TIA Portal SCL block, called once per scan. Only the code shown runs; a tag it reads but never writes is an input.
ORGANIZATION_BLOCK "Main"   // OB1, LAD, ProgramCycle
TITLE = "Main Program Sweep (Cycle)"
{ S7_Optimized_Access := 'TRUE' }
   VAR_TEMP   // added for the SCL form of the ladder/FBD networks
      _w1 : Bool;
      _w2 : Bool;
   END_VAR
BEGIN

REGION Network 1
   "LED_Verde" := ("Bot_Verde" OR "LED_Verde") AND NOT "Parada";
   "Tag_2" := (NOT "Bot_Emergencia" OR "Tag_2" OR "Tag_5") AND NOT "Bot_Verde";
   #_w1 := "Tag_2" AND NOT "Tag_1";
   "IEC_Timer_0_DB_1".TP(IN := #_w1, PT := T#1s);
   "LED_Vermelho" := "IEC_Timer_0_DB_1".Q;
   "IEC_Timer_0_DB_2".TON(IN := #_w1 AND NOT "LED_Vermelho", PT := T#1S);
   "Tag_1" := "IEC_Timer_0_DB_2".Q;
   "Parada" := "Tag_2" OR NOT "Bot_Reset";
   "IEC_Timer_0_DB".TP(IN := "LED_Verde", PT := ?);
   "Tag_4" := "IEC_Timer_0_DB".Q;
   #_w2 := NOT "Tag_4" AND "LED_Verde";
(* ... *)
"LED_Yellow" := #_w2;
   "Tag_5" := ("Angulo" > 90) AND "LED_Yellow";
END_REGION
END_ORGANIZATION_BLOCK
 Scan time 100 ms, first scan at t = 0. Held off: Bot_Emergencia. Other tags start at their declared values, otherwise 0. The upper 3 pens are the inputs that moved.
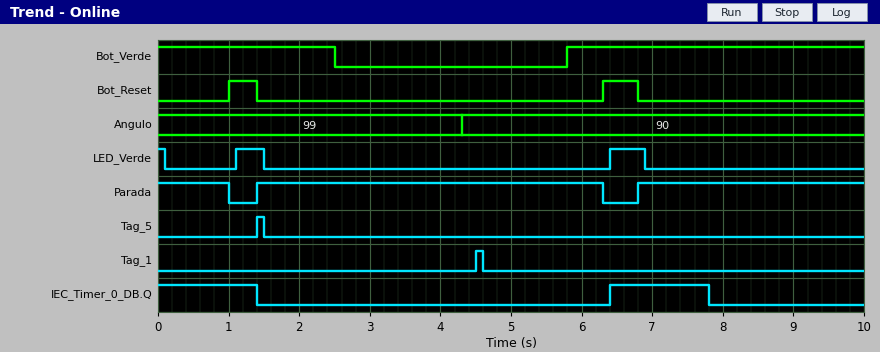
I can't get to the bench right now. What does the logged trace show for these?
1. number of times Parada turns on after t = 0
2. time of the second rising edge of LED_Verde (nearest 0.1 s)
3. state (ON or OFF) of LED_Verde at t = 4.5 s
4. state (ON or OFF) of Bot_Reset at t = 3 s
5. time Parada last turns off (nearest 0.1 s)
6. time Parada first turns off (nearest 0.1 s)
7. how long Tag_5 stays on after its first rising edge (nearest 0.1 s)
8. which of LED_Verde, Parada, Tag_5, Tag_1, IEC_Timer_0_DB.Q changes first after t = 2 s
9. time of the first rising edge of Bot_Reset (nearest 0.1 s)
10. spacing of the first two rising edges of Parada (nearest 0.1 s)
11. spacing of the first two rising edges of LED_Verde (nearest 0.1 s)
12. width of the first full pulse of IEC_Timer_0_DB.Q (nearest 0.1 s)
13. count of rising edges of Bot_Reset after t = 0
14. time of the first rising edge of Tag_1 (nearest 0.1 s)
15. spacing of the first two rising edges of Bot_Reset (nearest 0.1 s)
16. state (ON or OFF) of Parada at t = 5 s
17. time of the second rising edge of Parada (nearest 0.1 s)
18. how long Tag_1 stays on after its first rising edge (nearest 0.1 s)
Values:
2
6.4 s
OFF
OFF
6.3 s
1.0 s
0.1 s
Tag_1
1.0 s
5.4 s
5.3 s
1.4 s
2
4.5 s
5.3 s
ON
6.8 s
0.1 s
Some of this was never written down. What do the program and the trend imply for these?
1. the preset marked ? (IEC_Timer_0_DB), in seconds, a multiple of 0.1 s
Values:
1.4 s
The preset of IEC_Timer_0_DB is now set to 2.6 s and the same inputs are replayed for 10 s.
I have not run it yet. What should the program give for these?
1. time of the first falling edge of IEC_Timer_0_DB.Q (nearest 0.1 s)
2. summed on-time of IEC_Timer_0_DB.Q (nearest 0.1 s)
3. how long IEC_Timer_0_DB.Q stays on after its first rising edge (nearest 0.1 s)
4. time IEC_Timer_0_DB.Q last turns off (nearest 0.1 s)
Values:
2.6 s
5.2 s
2.6 s
9.0 s
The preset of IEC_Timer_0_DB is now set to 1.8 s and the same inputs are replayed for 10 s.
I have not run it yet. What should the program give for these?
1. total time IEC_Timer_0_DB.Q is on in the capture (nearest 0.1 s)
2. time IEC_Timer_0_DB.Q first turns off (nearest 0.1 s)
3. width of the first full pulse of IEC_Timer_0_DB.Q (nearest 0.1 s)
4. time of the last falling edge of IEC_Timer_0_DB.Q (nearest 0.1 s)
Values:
3.6 s
1.8 s
1.8 s
8.2 s
